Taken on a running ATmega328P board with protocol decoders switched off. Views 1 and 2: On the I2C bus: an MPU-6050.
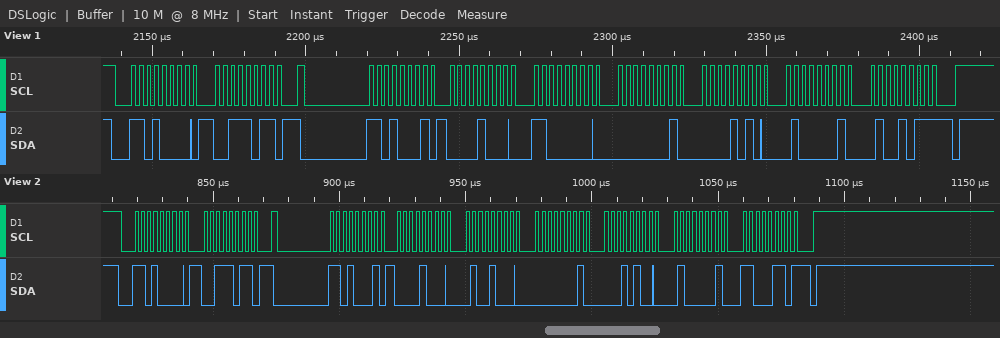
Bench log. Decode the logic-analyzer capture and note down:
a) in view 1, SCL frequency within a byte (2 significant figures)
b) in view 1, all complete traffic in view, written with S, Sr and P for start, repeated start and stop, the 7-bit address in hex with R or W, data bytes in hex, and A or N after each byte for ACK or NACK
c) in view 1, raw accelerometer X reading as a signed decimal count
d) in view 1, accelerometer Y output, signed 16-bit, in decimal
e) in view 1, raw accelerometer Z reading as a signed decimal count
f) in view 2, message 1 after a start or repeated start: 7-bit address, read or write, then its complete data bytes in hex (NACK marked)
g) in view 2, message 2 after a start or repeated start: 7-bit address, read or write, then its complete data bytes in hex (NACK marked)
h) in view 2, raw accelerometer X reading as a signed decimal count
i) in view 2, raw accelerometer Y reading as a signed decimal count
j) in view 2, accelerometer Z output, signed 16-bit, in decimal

400 kHz
S 68W A 3B A Sr 68R A 08 A C0 A 01 A 0A A 41 A 4B N P
2240
266
16715
0x68 write: 3B
0x68 read: 08 48 01 14 41 C6 NACK
2120
276
16838
